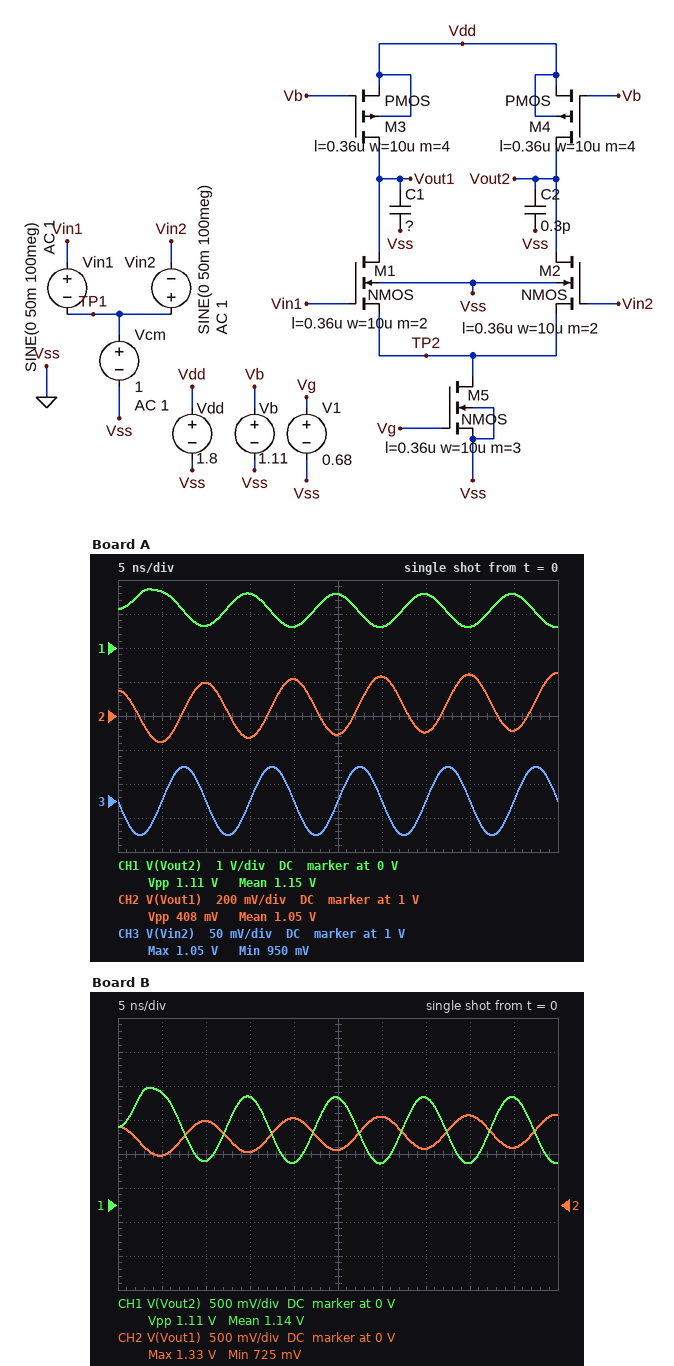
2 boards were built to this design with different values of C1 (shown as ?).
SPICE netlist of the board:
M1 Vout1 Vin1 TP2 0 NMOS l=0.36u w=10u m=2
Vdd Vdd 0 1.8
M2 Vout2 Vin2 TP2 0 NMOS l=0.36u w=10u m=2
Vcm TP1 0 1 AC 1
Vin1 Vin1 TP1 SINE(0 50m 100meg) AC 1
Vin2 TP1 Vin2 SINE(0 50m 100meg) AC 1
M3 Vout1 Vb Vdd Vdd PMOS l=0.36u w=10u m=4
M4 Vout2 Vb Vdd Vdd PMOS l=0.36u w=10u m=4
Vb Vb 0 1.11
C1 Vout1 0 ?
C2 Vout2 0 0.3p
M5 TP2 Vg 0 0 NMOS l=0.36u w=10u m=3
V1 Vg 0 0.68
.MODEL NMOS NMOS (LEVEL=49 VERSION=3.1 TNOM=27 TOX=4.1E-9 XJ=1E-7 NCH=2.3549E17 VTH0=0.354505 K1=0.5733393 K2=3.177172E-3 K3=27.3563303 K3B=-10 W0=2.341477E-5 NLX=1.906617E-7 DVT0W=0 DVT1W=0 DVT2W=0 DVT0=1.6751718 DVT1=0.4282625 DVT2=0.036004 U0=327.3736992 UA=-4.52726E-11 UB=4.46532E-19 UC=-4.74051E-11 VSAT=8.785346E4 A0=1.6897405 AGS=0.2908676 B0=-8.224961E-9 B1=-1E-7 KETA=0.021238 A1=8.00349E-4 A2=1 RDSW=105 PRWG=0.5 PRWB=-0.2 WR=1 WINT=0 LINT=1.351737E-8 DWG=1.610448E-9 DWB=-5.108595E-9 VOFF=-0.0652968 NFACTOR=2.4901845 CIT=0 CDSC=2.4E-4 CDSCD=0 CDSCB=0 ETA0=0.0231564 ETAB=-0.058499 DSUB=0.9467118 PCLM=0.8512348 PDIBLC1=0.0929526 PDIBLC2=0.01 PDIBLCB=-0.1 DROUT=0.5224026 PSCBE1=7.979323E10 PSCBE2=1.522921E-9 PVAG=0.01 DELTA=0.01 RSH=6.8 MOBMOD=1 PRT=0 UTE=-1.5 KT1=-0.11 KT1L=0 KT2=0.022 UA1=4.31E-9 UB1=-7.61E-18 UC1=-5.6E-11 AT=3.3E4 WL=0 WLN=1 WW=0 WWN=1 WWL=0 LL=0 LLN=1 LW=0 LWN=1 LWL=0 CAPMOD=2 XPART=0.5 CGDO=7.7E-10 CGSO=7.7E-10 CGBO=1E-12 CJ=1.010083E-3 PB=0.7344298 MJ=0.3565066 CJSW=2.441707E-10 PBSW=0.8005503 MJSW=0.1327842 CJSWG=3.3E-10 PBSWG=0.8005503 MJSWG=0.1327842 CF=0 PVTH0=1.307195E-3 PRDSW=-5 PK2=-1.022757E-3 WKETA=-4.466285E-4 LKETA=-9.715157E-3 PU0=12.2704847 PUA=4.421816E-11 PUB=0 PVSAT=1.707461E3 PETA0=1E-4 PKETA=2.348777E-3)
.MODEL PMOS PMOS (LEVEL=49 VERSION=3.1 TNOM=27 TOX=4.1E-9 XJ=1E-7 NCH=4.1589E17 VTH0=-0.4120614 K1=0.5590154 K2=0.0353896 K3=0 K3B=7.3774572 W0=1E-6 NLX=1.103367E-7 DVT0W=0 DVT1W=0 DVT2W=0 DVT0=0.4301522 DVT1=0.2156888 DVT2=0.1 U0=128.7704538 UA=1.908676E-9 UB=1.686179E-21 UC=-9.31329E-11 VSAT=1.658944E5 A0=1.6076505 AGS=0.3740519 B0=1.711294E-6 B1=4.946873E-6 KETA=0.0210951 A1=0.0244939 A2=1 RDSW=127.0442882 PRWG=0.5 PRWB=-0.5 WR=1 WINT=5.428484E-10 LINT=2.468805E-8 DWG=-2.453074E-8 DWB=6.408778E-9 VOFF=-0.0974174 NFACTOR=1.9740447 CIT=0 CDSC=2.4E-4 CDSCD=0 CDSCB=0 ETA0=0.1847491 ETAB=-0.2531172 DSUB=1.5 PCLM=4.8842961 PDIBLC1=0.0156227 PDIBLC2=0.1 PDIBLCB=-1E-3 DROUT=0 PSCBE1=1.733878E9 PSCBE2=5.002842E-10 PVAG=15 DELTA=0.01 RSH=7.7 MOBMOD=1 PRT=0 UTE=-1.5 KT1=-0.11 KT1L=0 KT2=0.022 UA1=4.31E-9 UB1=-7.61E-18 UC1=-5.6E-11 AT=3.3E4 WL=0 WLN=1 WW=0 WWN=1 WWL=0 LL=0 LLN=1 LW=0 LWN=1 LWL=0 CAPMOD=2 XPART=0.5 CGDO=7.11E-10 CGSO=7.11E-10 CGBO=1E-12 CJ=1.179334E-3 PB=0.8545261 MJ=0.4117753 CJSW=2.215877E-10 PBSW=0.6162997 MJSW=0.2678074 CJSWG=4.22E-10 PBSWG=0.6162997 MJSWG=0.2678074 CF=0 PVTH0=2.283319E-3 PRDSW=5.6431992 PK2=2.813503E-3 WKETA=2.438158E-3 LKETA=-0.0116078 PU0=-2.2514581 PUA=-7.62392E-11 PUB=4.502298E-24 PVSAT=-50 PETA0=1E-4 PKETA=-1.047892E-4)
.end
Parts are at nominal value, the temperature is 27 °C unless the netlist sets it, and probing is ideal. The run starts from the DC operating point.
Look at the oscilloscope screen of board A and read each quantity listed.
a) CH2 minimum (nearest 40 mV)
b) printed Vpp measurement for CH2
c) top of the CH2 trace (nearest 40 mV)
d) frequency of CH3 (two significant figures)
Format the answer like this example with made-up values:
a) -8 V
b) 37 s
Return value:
a) 840 mV
b) 408 mV
c) 1.24 V
d) 100 MHz
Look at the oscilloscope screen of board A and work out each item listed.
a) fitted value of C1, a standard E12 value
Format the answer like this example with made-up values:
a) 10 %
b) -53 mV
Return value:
a) 1 pF
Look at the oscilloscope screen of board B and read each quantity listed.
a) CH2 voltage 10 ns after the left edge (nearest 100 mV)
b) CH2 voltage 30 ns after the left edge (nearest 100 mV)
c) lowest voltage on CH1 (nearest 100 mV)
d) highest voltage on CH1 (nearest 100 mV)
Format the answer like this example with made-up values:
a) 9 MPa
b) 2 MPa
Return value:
a) 1.2 V
b) 1.3 V
c) 600 mV
d) 1.7 V
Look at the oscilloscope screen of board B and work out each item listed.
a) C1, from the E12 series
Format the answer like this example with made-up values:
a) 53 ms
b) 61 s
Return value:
a) 680 fF
